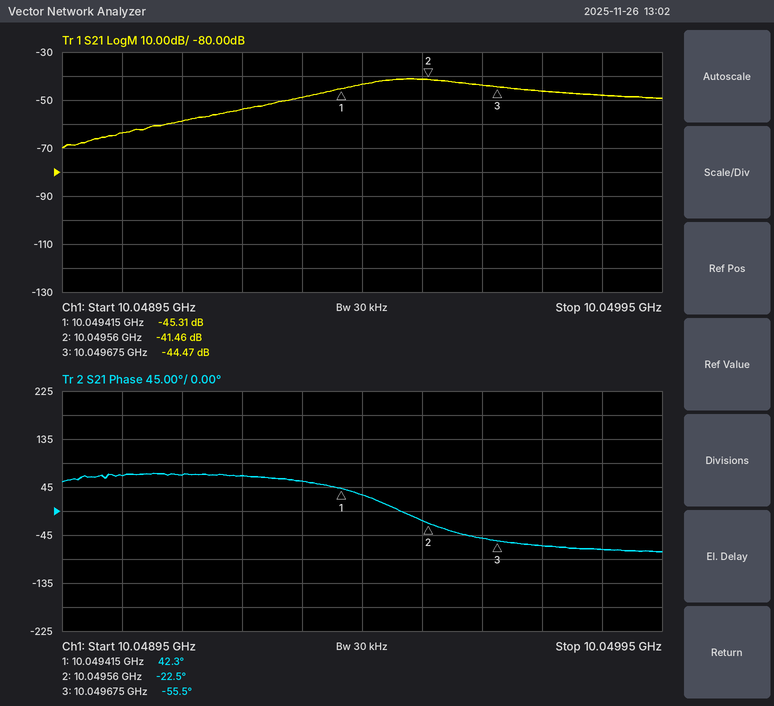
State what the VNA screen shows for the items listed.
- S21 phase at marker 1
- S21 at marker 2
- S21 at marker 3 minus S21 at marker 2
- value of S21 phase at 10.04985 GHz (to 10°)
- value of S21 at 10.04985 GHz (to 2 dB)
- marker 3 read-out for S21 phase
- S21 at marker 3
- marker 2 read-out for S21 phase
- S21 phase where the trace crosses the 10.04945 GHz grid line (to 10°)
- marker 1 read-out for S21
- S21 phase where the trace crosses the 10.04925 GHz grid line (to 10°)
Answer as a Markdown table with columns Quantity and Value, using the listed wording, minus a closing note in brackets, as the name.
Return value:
| Quantity | Value |
|---|---|
| S21 phase at marker 1 | 42.3° |
| S21 at marker 2 | -41.46 dB |
| S21 at marker 3 minus S21 at marker 2 | -3.01 dB |
| value of S21 phase at 10.04985 GHz | -70° |
| value of S21 at 10.04985 GHz | -48 dB |
| marker 3 read-out for S21 phase | -55.5° |
| S21 at marker 3 | -44.47 dB |
| marker 2 read-out for S21 phase | -22.5° |
| S21 phase where the trace crosses the 10.04945 GHz grid line | 30° |
| marker 1 read-out for S21 | -45.31 dB |
| S21 phase where the trace crosses the 10.04925 GHz grid line | 70° |
